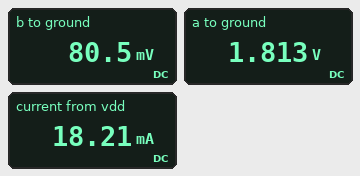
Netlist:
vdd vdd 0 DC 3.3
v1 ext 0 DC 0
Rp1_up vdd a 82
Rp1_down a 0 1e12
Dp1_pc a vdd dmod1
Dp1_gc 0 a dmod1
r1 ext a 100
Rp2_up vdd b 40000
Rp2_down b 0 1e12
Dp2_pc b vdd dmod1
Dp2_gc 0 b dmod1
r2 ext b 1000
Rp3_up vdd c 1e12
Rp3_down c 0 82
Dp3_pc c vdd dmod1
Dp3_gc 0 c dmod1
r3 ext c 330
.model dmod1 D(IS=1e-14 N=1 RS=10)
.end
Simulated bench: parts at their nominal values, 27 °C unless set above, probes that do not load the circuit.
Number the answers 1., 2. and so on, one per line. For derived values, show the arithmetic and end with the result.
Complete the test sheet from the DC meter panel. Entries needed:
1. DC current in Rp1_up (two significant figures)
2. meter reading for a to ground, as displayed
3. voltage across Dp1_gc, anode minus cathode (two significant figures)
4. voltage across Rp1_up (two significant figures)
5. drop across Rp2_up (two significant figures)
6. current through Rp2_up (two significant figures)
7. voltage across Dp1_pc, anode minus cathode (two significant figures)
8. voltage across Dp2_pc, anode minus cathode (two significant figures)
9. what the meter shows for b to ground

1. (3.3 V - 1.813 V) / 82 Ω = 18 mA
2. 1.813 V
3. 0 V - 1.813 V = -1.8 V
4. 3.3 V - 1.813 V = 1.5 V
5. 3.3 V - 80.5 mV = 3.2 V
6. (3.3 V - 80.5 mV) / 40 kΩ = 80 µA
7. 1.813 V - 3.3 V = -1.5 V
8. 80.5 mV - 3.3 V = -3.2 V
9. 80.5 mV
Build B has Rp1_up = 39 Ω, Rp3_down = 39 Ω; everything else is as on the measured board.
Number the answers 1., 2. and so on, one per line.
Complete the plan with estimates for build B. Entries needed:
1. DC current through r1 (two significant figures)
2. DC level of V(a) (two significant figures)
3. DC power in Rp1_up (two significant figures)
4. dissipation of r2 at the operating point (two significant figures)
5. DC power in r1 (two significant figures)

1. 24 mA
2. 2.4 V
3. 22 mW
4. 6.5 µW
5. 56 mW
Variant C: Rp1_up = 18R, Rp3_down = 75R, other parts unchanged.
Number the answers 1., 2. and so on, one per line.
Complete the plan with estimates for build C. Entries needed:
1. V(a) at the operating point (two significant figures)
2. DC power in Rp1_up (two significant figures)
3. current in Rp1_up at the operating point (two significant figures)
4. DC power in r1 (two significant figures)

1. 2.8 V
2. 14 mW
3. 28 mA
4. 78 mW
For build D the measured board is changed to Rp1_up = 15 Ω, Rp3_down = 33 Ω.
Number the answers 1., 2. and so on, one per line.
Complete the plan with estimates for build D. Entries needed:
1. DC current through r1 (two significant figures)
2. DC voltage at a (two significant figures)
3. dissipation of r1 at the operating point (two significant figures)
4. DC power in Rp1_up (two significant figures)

1. 29 mA
2. 2.9 V
3. 82 mW
4. 12 mW
